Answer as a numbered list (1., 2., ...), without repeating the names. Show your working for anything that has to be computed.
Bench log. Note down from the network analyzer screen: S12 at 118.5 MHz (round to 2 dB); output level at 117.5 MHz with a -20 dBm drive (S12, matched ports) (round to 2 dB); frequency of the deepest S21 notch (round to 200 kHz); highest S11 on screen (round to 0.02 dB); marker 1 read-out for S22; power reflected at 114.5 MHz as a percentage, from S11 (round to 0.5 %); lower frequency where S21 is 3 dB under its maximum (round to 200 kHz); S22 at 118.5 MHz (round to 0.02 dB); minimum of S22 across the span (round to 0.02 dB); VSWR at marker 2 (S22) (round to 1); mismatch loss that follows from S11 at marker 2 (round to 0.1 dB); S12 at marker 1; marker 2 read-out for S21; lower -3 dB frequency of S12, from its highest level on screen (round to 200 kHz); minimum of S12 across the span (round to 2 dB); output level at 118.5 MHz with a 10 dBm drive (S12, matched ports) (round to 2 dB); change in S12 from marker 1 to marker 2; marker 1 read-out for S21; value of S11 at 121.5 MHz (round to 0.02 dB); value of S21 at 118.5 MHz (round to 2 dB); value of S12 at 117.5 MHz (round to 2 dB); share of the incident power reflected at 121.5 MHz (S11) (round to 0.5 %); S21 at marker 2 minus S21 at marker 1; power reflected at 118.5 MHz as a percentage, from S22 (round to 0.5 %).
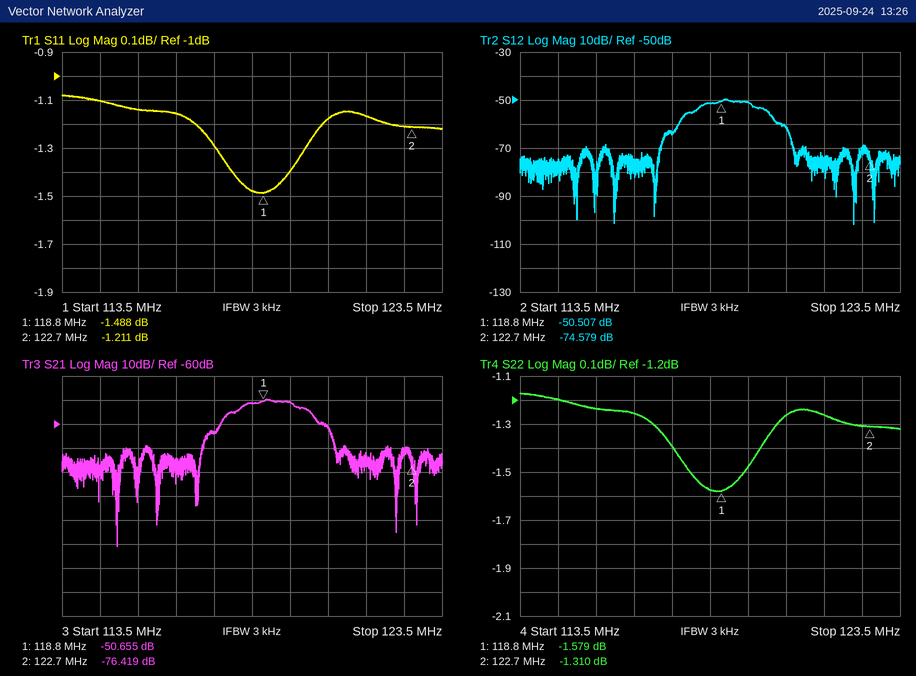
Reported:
1. -52 dB
2. -20 dBm + (-64 dB) = -84 dBm
3. 115.0 MHz
4. -1.08 dB
5. -1.579 dB
6. 10^(-1.1/10) ≈ 77.6 %, so 77.5 % to the nearest 0.5 %
7. 118.2 MHz
8. -1.58 dB
9. -1.58 dB
10. (1 + 0.8600)/(1 − 0.8600) ≈ 13
11. −10 log10(1 − 10^(-1.211/10)) ≈ 6.1 dB
12. -50.507 dB
13. -76.419 dB
14. 118.2 MHz
15. -102 dB
16. 10 dBm + (-52 dB) = -42 dBm
17. -74.579 − (-50.507) = -24.072 dB
18. -50.655 dB
19. -1.16 dB
20. -52 dB
21. -64 dB
22. 10^(-1.16/10) ≈ 76.6 %, so 76.5 % to the nearest 0.5 %
23. -76.419 − (-50.655) = -25.764 dB
24. 10^(-1.58/10) ≈ 69.5 %
